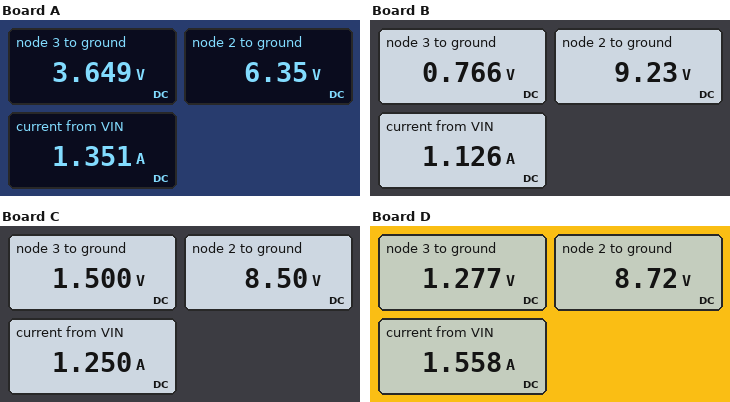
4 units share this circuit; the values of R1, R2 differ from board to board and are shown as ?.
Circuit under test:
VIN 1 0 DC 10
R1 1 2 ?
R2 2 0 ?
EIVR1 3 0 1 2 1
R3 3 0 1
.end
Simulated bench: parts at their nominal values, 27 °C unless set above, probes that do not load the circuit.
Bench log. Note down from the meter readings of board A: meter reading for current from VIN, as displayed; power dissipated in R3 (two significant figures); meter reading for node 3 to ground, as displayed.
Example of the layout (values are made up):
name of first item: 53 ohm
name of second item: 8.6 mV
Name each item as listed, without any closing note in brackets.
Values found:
meter reading for current from VIN, as displayed: 1.351 A
power dissipated in R3: 13 W
meter reading for node 3 to ground, as displayed: 3.649 V
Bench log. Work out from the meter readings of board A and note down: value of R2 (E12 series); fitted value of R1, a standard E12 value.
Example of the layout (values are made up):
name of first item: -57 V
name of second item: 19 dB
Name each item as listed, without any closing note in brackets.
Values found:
value of R2: 4.7 Ω
fitted value of R1, a standard E12 value: 2.7 Ω
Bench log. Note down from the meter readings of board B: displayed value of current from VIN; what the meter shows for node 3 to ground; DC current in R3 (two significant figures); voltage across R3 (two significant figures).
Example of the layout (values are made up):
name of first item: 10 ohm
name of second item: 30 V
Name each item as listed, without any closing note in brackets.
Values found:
displayed value of current from VIN: 1.126 A
what the meter shows for node 3 to ground: 0.766 V
DC current in R3: 770 mA
voltage across R3: 770 mV
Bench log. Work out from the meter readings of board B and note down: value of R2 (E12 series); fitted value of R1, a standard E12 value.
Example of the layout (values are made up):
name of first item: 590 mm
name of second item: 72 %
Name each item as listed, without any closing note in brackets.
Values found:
value of R2: 8.2 Ω
fitted value of R1, a standard E12 value: 0.68 Ω
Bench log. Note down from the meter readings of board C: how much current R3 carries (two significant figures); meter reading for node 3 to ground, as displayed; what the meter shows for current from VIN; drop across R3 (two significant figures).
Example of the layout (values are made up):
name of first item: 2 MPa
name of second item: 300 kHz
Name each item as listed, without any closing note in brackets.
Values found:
how much current R3 carries: 1.5 A
meter reading for node 3 to ground, as displayed: 1.500 V
what the meter shows for current from VIN: 1.250 A
drop across R3: 1.5 V
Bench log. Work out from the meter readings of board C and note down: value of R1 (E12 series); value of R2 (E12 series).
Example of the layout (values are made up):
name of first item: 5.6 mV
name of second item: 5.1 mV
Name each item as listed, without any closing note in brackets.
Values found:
value of R1: 1.2 Ω
value of R2: 6.8 Ω
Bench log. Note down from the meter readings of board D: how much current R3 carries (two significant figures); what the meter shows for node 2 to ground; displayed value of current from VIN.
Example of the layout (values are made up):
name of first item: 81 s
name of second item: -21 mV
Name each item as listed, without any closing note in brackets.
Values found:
how much current R3 carries: 1.3 A
what the meter shows for node 2 to ground: 8.72 V
displayed value of current from VIN: 1.558 A
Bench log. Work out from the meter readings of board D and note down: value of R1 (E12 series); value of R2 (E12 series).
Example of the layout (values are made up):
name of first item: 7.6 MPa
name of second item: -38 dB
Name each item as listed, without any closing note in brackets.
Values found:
value of R1: 0.82 Ω
value of R2: 5.6 Ω
